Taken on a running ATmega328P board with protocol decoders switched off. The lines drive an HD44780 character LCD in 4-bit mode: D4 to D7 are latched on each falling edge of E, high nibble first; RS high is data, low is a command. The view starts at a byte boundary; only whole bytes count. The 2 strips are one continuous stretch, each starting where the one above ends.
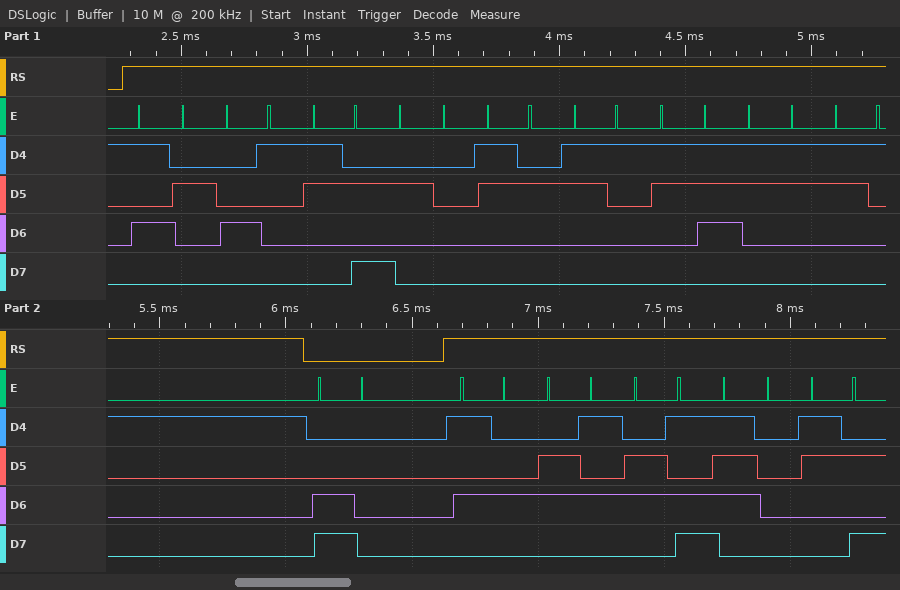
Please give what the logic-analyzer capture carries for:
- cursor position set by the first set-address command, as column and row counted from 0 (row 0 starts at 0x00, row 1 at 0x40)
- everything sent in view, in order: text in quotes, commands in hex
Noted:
column 0, row 1
"RA: 21731" 0xC0 "Temp:"
